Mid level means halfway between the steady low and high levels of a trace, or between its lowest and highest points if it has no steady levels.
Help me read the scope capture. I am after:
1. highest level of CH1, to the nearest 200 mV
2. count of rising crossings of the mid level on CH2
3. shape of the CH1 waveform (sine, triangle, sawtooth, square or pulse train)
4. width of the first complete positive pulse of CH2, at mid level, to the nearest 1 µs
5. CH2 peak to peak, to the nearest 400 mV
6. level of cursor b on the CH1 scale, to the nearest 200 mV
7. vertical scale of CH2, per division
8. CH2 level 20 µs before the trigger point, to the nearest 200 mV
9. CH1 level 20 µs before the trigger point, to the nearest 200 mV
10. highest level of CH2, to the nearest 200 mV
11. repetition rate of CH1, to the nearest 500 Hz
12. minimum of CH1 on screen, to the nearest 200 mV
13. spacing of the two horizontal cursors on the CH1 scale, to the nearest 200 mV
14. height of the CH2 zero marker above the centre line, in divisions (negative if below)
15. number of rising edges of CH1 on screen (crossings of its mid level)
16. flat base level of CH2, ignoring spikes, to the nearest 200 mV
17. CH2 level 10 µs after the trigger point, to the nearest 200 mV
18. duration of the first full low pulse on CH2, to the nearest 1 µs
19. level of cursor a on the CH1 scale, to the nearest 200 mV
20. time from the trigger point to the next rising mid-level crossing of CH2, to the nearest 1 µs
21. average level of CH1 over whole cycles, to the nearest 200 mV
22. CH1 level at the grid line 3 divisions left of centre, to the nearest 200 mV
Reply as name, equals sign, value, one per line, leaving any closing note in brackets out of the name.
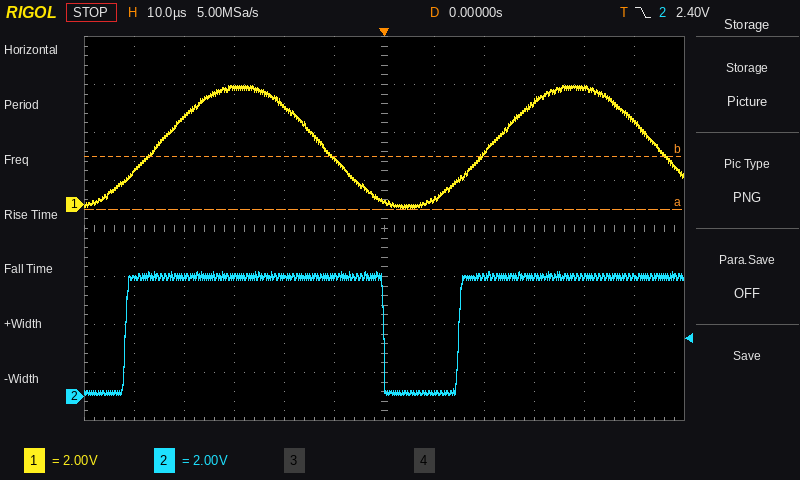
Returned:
highest level of CH1, to the nearest 200 mV = 5.0 V
count of rising crossings of the mid level on CH2 = 2
shape of the CH1 waveform = sine
width of the first complete positive pulse of CH2, at mid level, to the nearest 1 µs = 52 µs
CH2 peak to peak, to the nearest 400 mV = 5.2 V
level of cursor b on the CH1 scale, to the nearest 200 mV = 2.0 V
vertical scale of CH2, per division = 2 V
CH2 level 20 µs before the trigger point, to the nearest 200 mV = 5.0 V
CH1 level 20 µs before the trigger point, to the nearest 200 mV = 4.0 V
highest level of CH2, to the nearest 200 mV = 5.2 V
repetition rate of CH1, to the nearest 500 Hz = 15.0 kHz
minimum of CH1 on screen, to the nearest 200 mV = -200 mV
spacing of the two horizontal cursors on the CH1 scale, to the nearest 200 mV = 2.2 V
height of the CH2 zero marker above the centre line, in divisions = -3.5 div
number of rising edges of CH1 on screen = 2
flat base level of CH2, ignoring spikes, to the nearest 200 mV = 200 mV
CH2 level 10 µs after the trigger point, to the nearest 200 mV = 200 mV
duration of the first full low pulse on CH2, to the nearest 1 µs = 15 µs
level of cursor a on the CH1 scale, to the nearest 200 mV = -200 mV
time from the trigger point to the next rising mid-level crossing of CH2, to the nearest 1 µs = 15 µs
average level of CH1 over whole cycles, to the nearest 200 mV = 2.4 V
CH1 level at the grid line 3 divisions left of centre, to the nearest 200 mV = 4.8 V
